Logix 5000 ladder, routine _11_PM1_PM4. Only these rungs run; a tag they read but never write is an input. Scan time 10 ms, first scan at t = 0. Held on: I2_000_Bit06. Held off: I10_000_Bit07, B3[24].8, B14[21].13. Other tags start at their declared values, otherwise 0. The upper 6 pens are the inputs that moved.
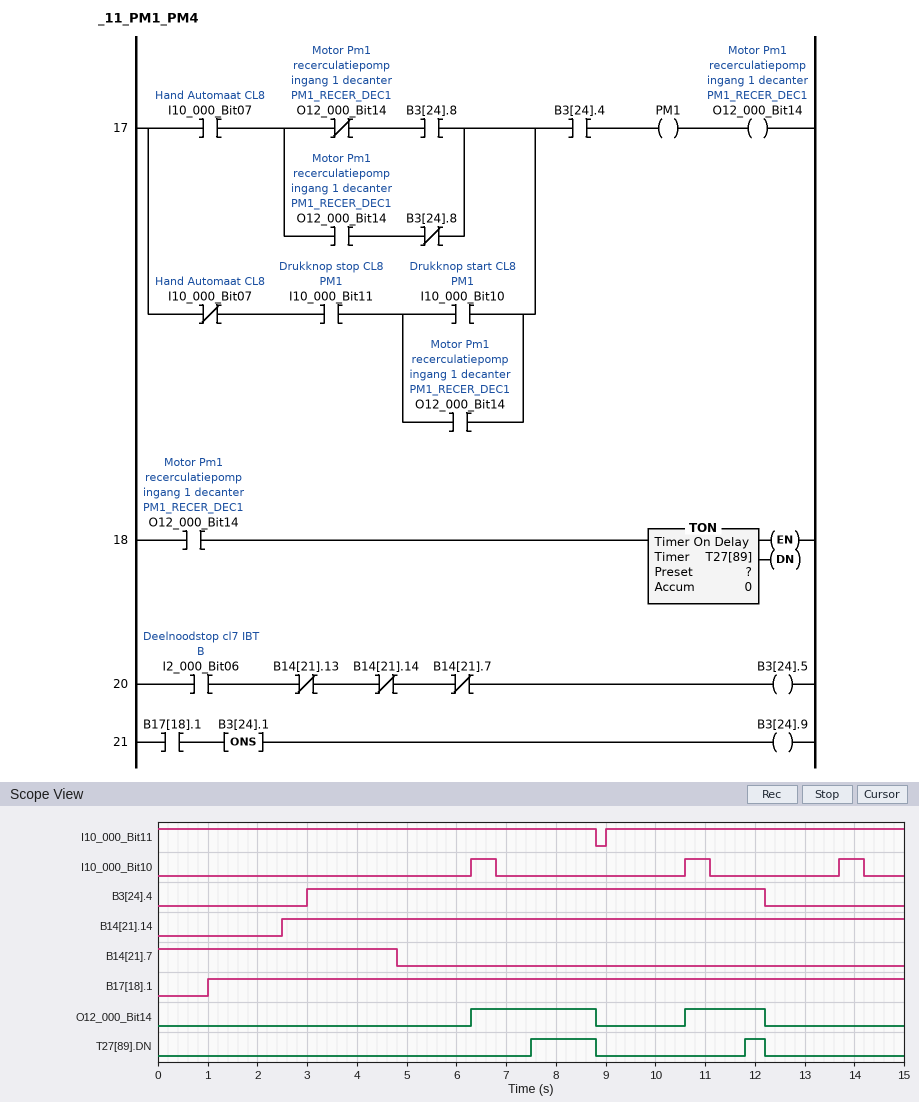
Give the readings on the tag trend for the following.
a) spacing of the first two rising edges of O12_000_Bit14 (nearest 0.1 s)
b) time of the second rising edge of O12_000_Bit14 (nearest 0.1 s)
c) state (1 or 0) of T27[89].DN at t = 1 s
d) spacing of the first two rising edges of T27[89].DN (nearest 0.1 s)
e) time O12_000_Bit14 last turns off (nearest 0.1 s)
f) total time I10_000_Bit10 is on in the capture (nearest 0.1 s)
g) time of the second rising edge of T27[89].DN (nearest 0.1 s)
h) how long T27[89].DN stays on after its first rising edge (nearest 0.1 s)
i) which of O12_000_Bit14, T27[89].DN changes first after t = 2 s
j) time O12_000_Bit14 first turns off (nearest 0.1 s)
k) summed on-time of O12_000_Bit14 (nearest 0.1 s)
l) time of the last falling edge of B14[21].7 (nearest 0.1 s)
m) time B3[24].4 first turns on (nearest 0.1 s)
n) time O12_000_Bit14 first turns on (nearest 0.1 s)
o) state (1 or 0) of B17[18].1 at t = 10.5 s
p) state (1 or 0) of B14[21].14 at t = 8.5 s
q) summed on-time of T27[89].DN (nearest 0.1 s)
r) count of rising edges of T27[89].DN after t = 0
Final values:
4.3 s
10.6 s
0
4.3 s
12.2 s
1.5 s
11.8 s
1.3 s
O12_000_Bit14
8.8 s
4.1 s
4.8 s
3.0 s
6.3 s
1
1
1.7 s
2
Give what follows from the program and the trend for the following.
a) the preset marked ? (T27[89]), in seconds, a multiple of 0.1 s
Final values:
1.2 s
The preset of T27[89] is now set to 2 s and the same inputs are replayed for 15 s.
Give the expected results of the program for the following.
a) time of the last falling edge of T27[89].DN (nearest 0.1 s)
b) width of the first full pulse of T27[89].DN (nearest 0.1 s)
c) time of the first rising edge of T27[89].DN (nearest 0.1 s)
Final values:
8.8 s
0.5 s
8.3 s
